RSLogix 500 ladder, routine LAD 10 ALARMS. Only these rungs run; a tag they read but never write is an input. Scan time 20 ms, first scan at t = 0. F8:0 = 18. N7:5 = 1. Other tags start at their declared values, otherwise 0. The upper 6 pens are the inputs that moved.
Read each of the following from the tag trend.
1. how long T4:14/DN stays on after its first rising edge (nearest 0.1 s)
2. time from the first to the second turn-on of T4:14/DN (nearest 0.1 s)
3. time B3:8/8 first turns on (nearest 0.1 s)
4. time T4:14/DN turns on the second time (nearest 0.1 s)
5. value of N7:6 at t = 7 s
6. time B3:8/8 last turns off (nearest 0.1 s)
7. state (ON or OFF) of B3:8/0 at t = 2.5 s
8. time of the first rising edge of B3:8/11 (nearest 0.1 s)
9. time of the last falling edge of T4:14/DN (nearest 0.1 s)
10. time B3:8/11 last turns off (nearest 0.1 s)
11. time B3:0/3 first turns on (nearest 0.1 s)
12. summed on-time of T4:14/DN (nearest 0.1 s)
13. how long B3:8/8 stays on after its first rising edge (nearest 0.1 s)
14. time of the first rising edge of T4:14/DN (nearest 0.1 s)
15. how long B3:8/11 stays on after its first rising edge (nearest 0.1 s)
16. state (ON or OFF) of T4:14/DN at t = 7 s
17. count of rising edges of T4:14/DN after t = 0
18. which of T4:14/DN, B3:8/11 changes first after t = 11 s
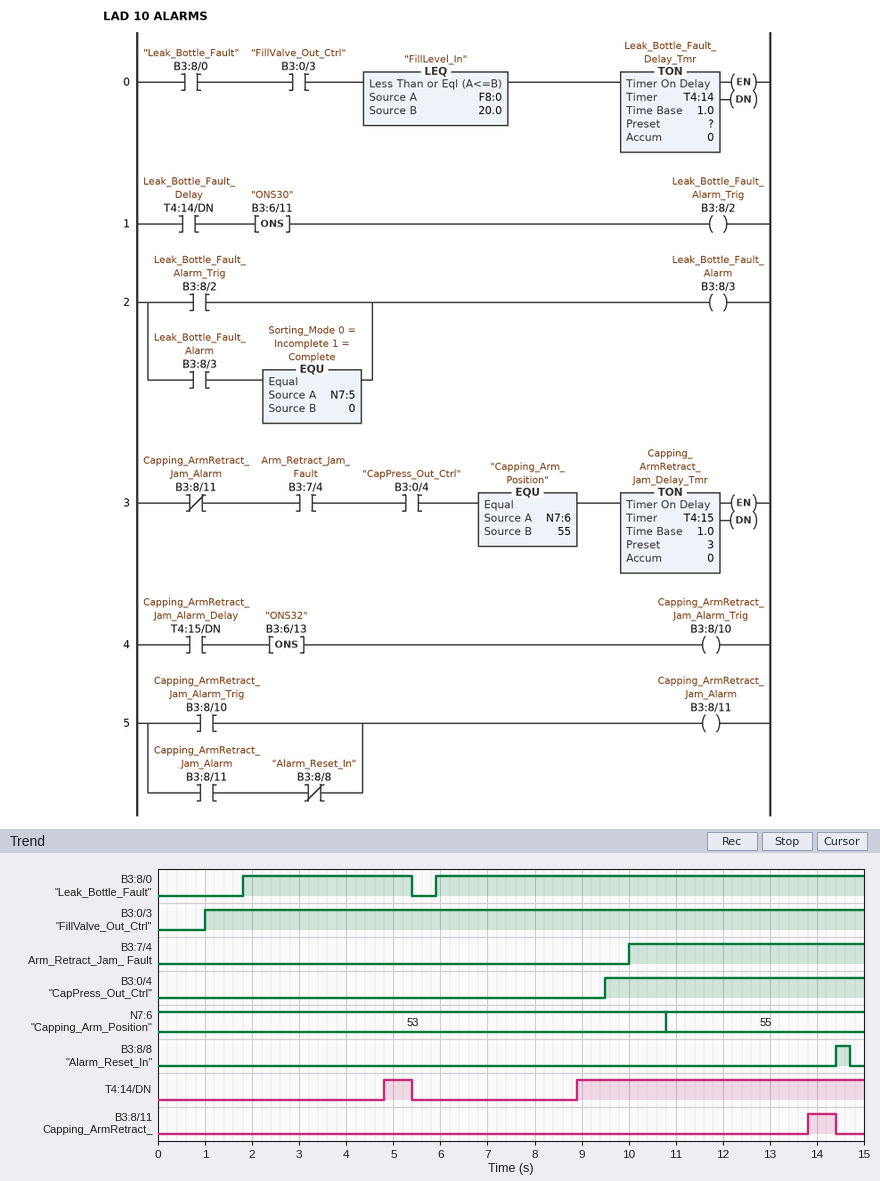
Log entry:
0.6 s
4.1 s
14.4 s
8.9 s
53
14.7 s
ON
13.8 s
5.4 s
14.4 s
1.0 s
6.7 s
0.3 s
4.8 s
0.6 s
OFF
2
B3:8/11
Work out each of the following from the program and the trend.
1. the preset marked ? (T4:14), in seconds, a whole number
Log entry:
3 s
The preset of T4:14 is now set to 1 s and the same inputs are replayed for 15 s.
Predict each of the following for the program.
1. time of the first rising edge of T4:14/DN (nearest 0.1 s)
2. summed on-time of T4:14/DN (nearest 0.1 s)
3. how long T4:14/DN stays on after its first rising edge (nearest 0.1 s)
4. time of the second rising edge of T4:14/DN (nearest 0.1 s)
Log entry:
2.8 s
10.7 s
2.6 s
6.9 s
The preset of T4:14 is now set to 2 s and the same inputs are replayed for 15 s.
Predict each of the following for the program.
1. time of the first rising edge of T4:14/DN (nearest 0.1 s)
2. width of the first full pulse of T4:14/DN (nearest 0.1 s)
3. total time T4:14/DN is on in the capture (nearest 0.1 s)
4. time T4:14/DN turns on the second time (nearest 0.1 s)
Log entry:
3.8 s
1.6 s
8.7 s
7.9 s
